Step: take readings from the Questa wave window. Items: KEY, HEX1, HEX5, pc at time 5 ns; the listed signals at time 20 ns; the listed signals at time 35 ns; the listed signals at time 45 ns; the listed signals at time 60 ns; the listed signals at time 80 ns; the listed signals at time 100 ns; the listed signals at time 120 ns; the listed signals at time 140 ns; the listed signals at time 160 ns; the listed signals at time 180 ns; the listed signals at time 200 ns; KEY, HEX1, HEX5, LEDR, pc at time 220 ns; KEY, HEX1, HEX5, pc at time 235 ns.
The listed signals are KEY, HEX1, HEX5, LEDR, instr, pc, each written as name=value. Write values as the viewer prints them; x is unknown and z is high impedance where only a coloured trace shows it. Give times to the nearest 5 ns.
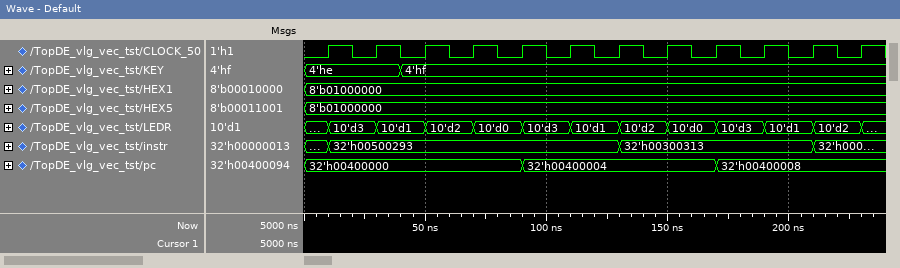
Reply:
KEY=4'he, HEX1=8'b01000000, HEX5=8'b01000000, pc=32'h00400000
KEY=4'he, HEX1=8'b01000000, HEX5=8'b01000000, LEDR=10'd3, instr=32'h00500293, pc=32'h00400000
KEY=4'he, HEX1=8'b01000000, HEX5=8'b01000000, LEDR=10'd1, instr=32'h00500293, pc=32'h00400000
KEY=4'hf, HEX1=8'b01000000, HEX5=8'b01000000, LEDR=10'd1, instr=32'h00500293, pc=32'h00400000
KEY=4'hf, HEX1=8'b01000000, HEX5=8'b01000000, LEDR=10'd2, instr=32'h00500293, pc=32'h00400000
KEY=4'hf, HEX1=8'b01000000, HEX5=8'b01000000, LEDR=10'd0, instr=32'h00500293, pc=32'h00400000
KEY=4'hf, HEX1=8'b01000000, HEX5=8'b01000000, LEDR=10'd3, instr=32'h00500293, pc=32'h00400004
KEY=4'hf, HEX1=8'b01000000, HEX5=8'b01000000, LEDR=10'd1, instr=32'h00500293, pc=32'h00400004
KEY=4'hf, HEX1=8'b01000000, HEX5=8'b01000000, LEDR=10'd2, instr=32'h00300313, pc=32'h00400004
KEY=4'hf, HEX1=8'b01000000, HEX5=8'b01000000, LEDR=10'd0, instr=32'h00300313, pc=32'h00400004
KEY=4'hf, HEX1=8'b01000000, HEX5=8'b01000000, LEDR=10'd3, instr=32'h00300313, pc=32'h00400008
KEY=4'hf, HEX1=8'b01000000, HEX5=8'b01000000, LEDR=10'd1, instr=32'h00300313, pc=32'h00400008
KEY=4'hf, HEX1=8'b01000000, HEX5=8'b01000000, LEDR=10'd2, pc=32'h00400008
KEY=4'hf, HEX1=8'b01000000, HEX5=8'b01000000, pc=32'h00400008
